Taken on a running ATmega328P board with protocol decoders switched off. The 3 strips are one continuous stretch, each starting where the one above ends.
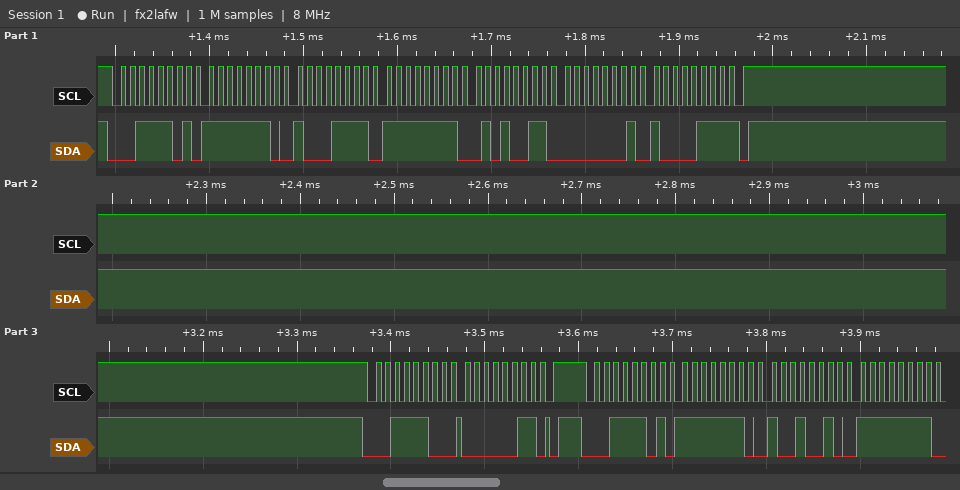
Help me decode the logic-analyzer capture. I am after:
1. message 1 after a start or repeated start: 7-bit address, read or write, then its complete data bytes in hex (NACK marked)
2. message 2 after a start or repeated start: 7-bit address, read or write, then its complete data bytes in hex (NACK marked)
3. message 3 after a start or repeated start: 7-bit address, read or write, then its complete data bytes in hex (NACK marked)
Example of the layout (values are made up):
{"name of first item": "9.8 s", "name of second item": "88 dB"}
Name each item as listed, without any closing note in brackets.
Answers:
{"message 1 after a start or repeated start: 7-bit address, read or write, then its complete data bytes in hex": "0x1E read: FE 8F FF 53 01 87 NACK", "message 2 after a start or repeated start: 7-bit address, read or write, then its complete data bytes in hex": "0x1E write: 03", "message 3 after a start or repeated start: 7-bit address, read or write, then its complete data bytes in hex": "0x1E read: FE 92 FF"}
